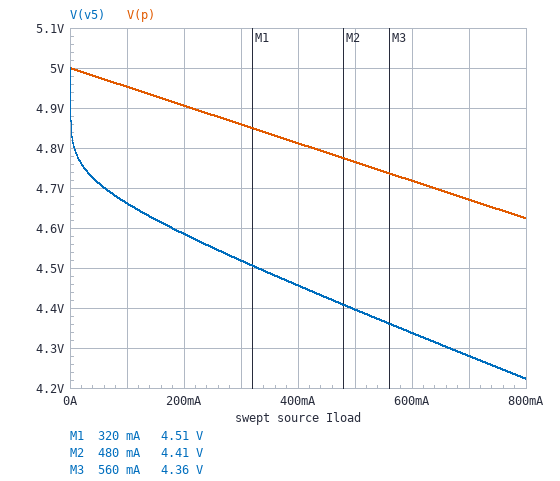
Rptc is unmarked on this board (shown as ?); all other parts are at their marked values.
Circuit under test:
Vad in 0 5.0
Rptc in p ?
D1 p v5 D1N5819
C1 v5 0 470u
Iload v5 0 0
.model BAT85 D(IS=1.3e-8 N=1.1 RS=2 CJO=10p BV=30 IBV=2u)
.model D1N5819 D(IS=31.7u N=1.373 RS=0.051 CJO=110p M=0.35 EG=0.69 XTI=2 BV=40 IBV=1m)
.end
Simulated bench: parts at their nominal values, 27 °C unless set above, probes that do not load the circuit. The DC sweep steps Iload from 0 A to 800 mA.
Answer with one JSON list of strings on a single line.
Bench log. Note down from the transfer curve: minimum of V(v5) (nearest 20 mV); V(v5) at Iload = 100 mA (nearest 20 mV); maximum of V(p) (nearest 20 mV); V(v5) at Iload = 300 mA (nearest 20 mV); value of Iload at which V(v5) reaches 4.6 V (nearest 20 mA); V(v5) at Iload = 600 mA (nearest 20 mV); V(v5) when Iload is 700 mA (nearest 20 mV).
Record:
["4.22 V", "4.66 V", "5.00 V", "4.52 V", "180 mA", "4.34 V", "4.28 V"]
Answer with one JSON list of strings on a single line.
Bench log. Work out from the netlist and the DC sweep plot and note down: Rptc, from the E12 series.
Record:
["0.47 Ω"]
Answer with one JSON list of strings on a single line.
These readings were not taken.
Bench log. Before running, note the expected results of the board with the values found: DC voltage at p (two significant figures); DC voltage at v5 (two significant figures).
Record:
["5.0 V", "5.0 V"]
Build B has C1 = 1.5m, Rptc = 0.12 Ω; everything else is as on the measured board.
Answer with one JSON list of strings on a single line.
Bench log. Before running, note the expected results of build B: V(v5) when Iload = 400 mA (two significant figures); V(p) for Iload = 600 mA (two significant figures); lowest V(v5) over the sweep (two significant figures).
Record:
["4.6 V", "4.9 V", "4.5 V"]
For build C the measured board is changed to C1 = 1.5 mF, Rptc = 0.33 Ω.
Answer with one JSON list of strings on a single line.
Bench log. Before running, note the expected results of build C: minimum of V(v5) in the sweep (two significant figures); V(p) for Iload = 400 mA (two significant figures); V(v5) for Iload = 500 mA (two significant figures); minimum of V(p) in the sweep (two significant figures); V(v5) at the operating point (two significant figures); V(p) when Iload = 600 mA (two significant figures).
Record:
["4.3 V", "4.9 V", "4.5 V", "4.7 V", "5.0 V", "4.8 V"]
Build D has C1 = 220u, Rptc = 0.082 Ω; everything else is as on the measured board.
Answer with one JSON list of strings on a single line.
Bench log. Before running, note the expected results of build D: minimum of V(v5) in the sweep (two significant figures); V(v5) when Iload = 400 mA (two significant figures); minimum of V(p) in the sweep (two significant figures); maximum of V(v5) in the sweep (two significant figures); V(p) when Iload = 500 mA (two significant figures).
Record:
["4.5 V", "4.6 V", "4.9 V", "5.0 V", "5.0 V"]
